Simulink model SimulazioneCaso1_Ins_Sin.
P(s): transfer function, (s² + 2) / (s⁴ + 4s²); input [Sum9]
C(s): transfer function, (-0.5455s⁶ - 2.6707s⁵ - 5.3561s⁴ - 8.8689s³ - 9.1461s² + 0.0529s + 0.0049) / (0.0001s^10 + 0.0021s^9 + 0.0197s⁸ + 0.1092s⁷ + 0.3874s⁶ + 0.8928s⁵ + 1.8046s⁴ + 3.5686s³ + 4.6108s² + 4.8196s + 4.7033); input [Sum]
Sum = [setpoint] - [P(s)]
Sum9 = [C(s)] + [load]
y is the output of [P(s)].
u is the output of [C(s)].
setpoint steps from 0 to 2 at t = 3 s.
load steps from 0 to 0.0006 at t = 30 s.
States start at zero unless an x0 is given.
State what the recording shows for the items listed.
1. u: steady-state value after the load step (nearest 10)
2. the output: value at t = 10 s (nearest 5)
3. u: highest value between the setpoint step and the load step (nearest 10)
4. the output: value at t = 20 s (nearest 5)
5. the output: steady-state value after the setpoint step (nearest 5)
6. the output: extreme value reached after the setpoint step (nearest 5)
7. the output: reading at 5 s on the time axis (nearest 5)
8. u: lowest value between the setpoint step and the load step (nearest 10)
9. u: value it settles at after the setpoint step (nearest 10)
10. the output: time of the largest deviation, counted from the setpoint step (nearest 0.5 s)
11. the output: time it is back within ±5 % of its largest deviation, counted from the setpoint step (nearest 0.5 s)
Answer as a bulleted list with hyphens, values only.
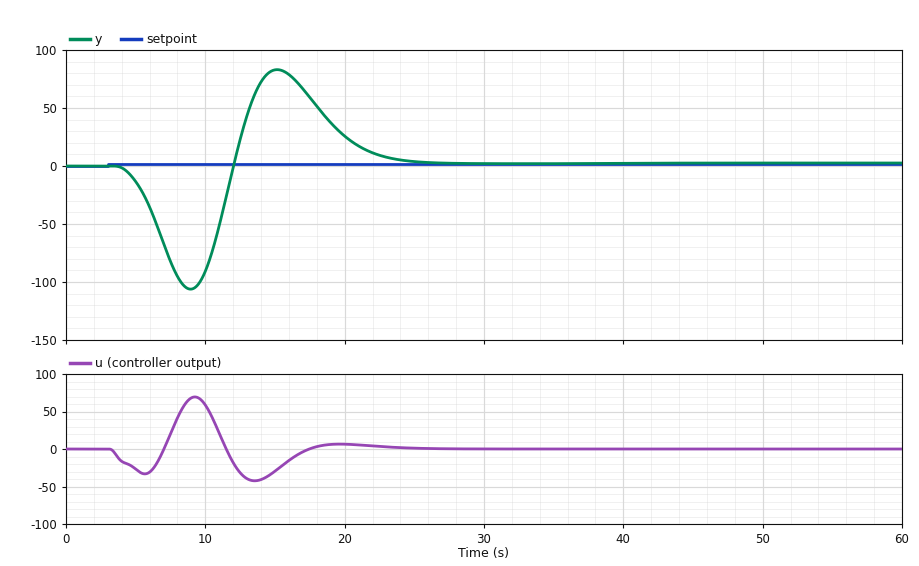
- 0
- -90
- 70
- 25
- 0
- -105
- -15
- -40
- 0
- 6.0 s
- 20.0 s
